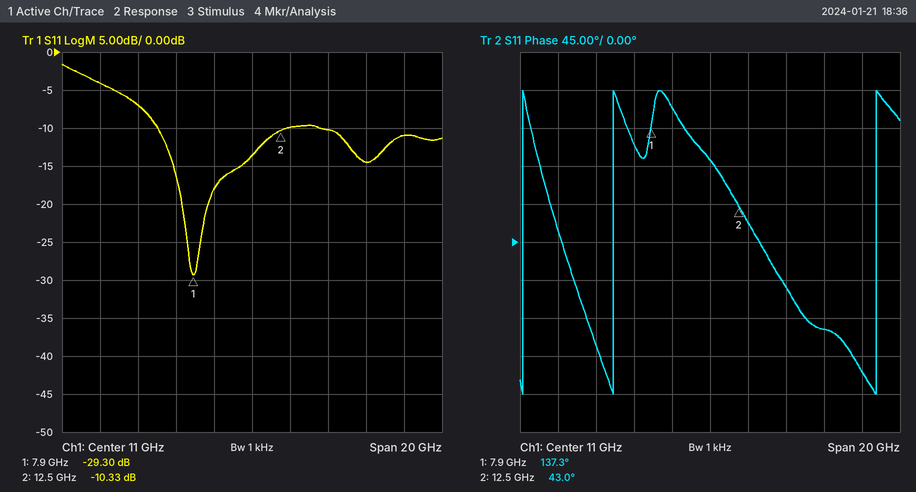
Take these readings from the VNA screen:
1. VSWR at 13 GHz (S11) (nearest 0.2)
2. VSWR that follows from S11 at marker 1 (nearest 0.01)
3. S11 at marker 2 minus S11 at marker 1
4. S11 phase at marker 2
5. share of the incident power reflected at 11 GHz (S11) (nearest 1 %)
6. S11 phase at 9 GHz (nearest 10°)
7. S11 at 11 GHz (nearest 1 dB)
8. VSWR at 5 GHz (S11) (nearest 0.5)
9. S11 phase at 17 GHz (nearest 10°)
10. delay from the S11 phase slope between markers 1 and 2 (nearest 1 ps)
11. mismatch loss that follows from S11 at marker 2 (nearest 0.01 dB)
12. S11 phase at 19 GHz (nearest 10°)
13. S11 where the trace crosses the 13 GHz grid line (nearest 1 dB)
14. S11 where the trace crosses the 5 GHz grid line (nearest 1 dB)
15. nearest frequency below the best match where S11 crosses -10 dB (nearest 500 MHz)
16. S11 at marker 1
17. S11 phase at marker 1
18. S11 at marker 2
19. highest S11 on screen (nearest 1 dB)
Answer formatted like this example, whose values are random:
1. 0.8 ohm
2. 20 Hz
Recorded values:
1. 2.0
2. 1.07
3. 18.97 dB
4. 43.0°
5. 4 %
6. 160°
7. -14 dB
8. 2.5
9. -100°
10. 57 ps
11. 0.42 dB
12. -150°
13. -10 dB
14. -7 dB
15. 6.0 GHz
16. -29.30 dB
17. 137.3°
18. -10.33 dB
19. -2 dB
